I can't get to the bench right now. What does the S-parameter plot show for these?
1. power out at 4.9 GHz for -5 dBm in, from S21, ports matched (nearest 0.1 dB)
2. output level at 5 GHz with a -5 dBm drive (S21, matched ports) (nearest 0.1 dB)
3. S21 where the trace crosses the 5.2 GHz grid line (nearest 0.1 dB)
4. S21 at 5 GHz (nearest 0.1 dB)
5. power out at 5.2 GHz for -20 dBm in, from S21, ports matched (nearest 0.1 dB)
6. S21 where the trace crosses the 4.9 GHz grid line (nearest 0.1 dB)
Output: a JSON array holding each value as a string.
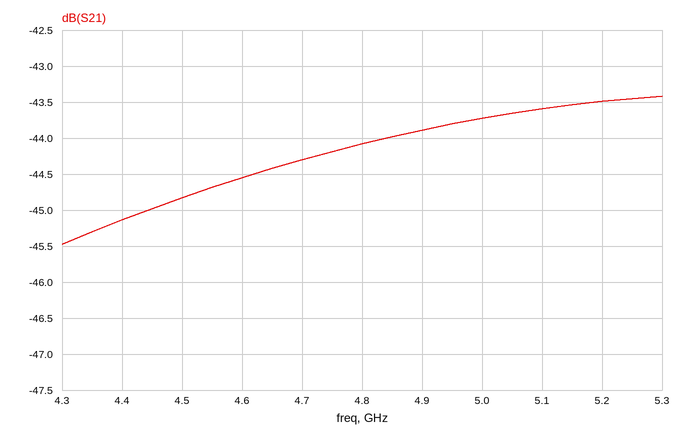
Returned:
["-48.9 dBm", "-48.7 dBm", "-43.5 dB", "-43.7 dB", "-63.5 dBm", "-43.9 dB"]
